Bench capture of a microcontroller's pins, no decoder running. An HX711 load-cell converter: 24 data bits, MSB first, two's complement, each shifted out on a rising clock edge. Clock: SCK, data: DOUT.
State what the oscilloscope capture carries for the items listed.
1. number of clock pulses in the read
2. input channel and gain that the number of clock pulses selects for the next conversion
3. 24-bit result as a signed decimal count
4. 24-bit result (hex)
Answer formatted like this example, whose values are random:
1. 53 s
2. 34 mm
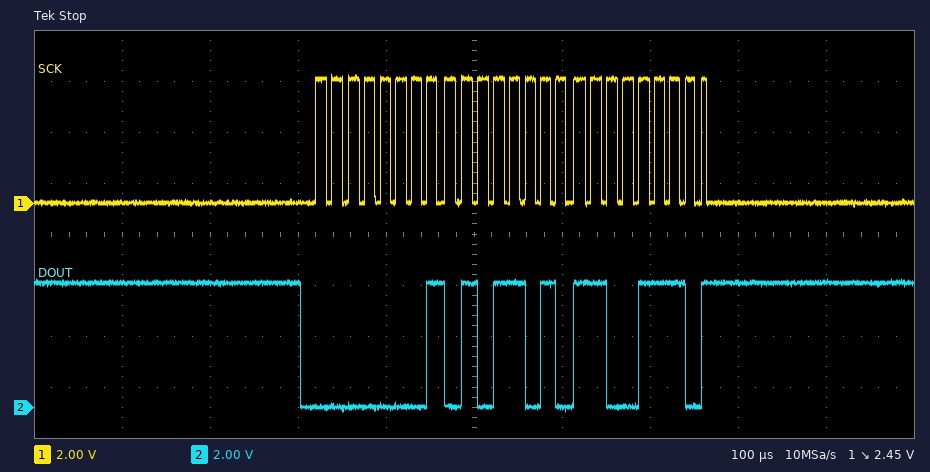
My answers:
1. 25
2. channel A, gain 128
3. 88782
4. 0x015ACE
